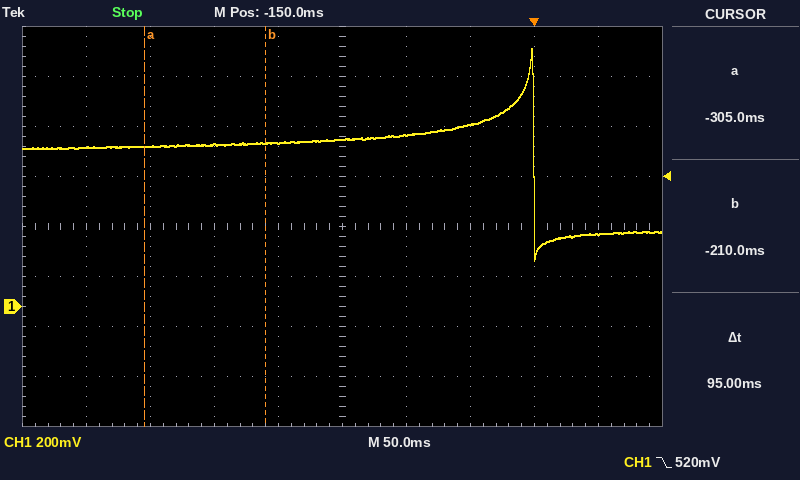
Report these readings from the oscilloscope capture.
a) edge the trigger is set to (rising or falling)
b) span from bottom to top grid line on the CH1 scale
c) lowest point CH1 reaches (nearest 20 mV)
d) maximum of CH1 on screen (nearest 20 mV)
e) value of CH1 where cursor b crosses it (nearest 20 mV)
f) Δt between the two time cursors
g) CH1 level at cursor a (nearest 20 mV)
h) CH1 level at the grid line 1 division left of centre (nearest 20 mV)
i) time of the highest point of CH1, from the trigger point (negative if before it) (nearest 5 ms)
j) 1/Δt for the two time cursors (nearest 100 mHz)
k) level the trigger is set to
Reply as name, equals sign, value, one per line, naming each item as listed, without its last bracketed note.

edge the trigger is set to = falling
span from bottom to top grid line on the CH1 scale = 1.6 V
lowest point CH1 reaches = 180 mV
maximum of CH1 on screen = 1.04 V
value of CH1 where cursor b crosses it = 660 mV
Δt between the two time cursors = 95 ms
CH1 level at cursor a = 640 mV
CH1 level at the grid line 1 division left of centre = 660 mV
time of the highest point of CH1, from the trigger point (negative if before it) = 0 ms
1/Δt for the two time cursors = 10.5 Hz
level the trigger is set to = 520 mV
